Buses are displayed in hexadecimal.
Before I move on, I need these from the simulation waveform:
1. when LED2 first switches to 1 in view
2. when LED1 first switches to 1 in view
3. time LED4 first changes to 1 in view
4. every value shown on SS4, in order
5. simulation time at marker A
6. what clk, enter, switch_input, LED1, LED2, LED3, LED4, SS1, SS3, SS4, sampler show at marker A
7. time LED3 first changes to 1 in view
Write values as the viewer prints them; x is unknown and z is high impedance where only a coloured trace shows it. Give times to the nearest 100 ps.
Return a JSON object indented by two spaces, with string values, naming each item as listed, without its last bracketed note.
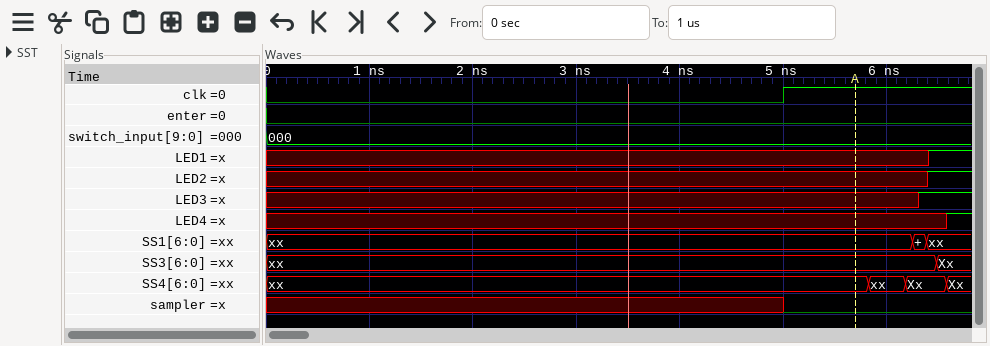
{
  "when LED2 first switches to 1 in view": "6400 ps",
  "when LED1 first switches to 1 in view": "6400 ps",
  "time LED4 first changes to 1 in view": "6600 ps",
  "every value shown on SS4, in order": "xx, xx, Xx, Xx",
  "simulation time at marker A": "5700 ps",
  "what clk, enter, switch_input, LED1, LED2, LED3, LED4, SS1, SS3, SS4, sampler show at marker A": "clk=1, enter=0, switch_input=000, LED1=x, LED2=x, LED3=x, LED4=x, SS1=xx, SS3=xx, SS4=xx, sampler=0",
  "time LED3 first changes to 1 in view": "6300 ps"
}
